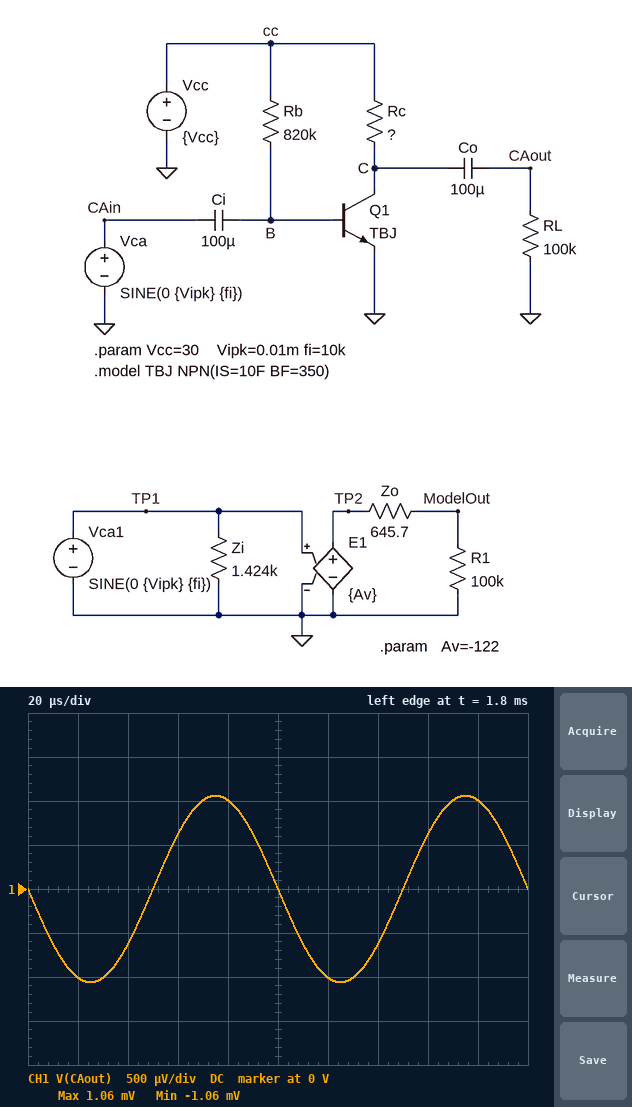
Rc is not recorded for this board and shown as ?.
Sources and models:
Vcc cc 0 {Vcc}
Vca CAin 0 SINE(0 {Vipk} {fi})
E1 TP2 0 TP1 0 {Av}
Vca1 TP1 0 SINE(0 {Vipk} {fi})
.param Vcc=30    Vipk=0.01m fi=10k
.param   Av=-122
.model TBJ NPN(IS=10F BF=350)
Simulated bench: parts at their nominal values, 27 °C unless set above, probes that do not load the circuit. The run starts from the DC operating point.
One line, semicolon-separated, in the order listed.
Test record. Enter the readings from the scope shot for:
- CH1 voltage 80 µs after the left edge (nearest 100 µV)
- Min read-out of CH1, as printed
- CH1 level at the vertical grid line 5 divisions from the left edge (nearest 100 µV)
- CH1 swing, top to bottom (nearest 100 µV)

1.0 mV; -1.06 mV; 0 V; 2.1 mV
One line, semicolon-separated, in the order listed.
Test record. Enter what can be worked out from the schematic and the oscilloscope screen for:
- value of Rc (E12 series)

220 Ω
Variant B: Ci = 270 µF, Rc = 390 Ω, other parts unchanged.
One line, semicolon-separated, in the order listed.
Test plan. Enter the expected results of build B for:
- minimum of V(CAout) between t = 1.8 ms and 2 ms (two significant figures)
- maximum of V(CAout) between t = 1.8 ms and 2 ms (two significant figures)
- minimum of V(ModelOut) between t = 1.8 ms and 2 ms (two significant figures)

-1.9 mV; 1.9 mV; -1.2 mV
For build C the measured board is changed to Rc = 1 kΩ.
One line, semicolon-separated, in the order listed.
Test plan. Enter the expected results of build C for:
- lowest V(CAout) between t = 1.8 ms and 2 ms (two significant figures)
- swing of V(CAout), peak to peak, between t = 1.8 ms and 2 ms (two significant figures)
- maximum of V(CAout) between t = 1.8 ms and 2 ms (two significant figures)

-4.8 mV; 9.6 mV; 4.8 mV
